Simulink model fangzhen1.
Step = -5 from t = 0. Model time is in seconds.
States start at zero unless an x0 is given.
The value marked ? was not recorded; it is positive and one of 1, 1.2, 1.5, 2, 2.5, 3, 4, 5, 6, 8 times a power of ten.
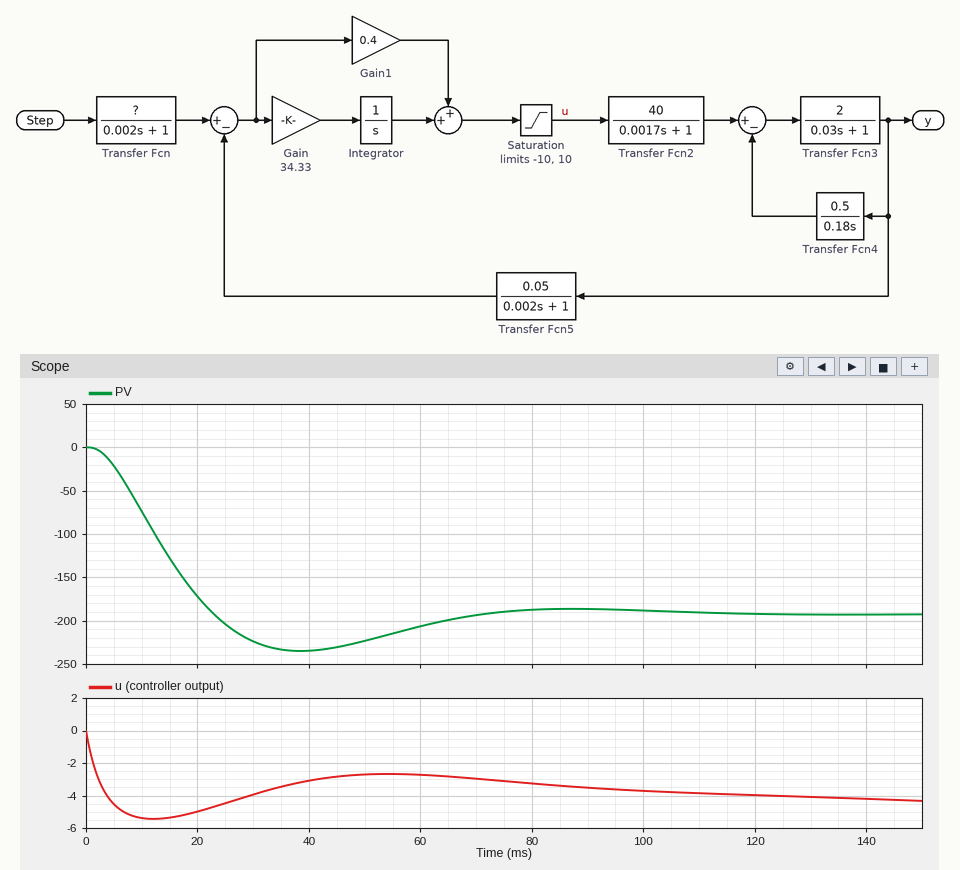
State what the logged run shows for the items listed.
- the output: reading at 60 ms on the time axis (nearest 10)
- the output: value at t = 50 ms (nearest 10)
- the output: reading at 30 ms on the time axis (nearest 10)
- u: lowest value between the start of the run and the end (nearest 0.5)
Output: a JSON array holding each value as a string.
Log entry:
["-210", "-220", "-220", "-5.5"]
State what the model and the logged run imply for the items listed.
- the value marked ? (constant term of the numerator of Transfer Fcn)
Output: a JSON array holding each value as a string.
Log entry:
["2"]
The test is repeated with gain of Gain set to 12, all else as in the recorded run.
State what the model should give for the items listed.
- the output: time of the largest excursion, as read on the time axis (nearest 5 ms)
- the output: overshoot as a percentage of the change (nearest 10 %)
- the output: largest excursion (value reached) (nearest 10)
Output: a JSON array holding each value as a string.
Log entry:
["75 ms", "70 %", "-180"]
